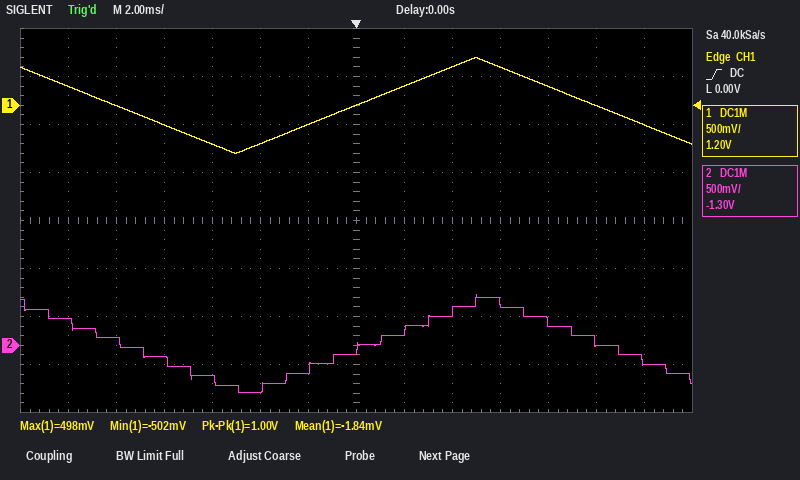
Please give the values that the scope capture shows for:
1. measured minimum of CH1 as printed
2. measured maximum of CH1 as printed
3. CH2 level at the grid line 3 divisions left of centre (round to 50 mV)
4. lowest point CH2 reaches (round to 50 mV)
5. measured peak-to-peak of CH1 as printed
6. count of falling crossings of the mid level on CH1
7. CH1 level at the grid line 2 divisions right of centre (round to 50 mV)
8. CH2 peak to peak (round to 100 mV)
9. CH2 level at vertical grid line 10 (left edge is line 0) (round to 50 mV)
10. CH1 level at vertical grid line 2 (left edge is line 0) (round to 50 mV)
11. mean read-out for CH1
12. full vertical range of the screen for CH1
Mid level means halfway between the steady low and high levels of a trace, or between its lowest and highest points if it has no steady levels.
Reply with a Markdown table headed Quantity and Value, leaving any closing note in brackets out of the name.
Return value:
| Quantity | Value |
|---|---|
| measured minimum of CH1 as printed | -502 mV |
| measured maximum of CH1 as printed | 498 mV |
| CH2 level at the grid line 3 divisions left of centre | -300 mV |
| lowest point CH2 reaches | -500 mV |
| measured peak-to-peak of CH1 as printed | 1.00 V |
| count of falling crossings of the mid level on CH1 | 2 |
| CH1 level at the grid line 2 divisions right of centre | 400 mV |
| CH2 peak to peak | 1.00 V |
| CH2 level at vertical grid line 10 (left edge is line 0) | 450 mV |
| CH1 level at vertical grid line 2 (left edge is line 0) | 0 mV |
| mean read-out for CH1 | -1.84 mV |
| full vertical range of the screen for CH1 | 4 V |
